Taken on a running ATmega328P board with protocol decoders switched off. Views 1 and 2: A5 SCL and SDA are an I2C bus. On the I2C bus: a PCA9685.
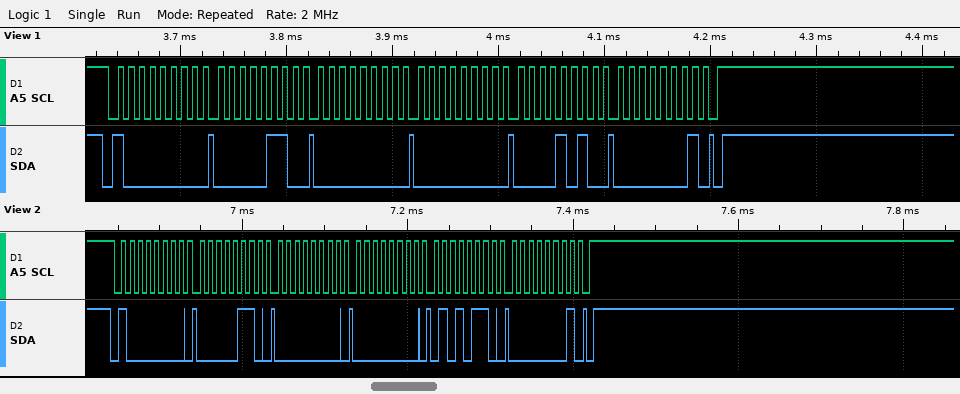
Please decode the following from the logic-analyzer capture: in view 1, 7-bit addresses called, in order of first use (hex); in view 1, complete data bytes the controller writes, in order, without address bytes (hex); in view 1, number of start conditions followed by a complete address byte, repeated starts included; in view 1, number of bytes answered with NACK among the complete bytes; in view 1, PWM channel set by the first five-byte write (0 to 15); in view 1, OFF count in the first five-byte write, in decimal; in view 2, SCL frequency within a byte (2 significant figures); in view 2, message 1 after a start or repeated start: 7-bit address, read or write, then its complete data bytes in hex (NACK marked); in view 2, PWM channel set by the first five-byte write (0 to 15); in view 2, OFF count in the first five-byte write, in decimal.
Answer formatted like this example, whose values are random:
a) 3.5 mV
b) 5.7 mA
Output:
a) 0x40
b) 06 00 00 0A 01
c) 1
d) 0
e) 0
f) 266
g) 100 kHz
h) 0x40 write: 06 00 00 56 01
i) 0
j) 342
